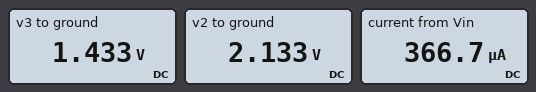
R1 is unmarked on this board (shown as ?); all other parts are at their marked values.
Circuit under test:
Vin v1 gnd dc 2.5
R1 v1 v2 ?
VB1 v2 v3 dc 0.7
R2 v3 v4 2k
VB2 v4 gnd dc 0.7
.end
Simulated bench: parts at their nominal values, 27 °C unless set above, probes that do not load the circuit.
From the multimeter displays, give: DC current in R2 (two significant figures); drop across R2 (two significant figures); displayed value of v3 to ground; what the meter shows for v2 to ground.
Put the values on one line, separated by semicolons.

370 µA; 730 mV; 1.433 V; 2.133 V
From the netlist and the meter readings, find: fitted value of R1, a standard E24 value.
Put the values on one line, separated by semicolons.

1 kΩ
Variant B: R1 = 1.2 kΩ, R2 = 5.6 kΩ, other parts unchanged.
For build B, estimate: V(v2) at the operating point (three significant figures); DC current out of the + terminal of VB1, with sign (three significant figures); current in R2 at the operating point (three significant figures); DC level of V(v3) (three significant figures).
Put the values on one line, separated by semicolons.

2.31 V; -162 µA; 162 µA; 1.61 V
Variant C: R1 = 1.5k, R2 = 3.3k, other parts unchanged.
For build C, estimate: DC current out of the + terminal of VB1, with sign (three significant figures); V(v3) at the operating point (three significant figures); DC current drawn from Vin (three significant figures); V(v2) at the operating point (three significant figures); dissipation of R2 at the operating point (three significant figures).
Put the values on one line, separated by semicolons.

-229 µA; 1.46 V; 229 µA; 2.16 V; 173 µW
